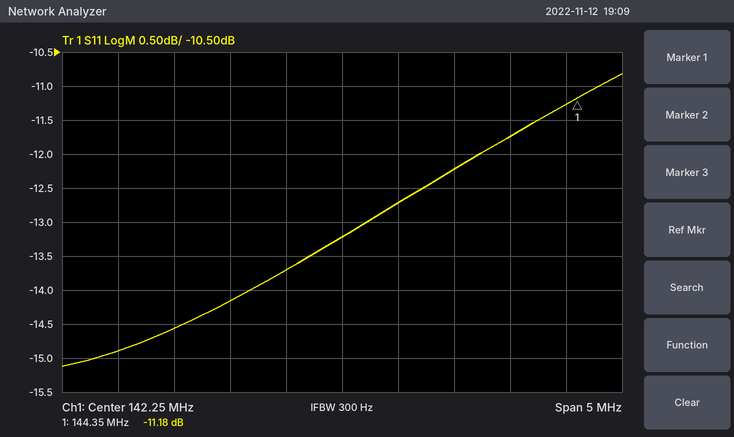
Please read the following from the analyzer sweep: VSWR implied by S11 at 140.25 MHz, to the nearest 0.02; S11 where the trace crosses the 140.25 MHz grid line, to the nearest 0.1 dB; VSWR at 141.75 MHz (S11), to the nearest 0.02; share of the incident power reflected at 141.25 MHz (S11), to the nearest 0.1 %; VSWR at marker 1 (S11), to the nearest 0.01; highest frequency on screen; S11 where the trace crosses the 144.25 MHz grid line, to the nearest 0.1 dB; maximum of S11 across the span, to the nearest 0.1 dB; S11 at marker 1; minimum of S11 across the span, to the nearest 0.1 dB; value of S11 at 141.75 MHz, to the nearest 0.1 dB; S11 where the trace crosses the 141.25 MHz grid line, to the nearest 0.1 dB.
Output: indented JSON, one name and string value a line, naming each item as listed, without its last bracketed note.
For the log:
{
  "VSWR implied by S11 at 140.25 MHz, to the nearest 0.02": "1.44",
  "S11 where the trace crosses the 140.25 MHz grid line, to the nearest 0.1 dB": "-14.9 dB",
  "VSWR at 141.75 MHz (S11), to the nearest 0.02": "1.52",
  "share of the incident power reflected at 141.25 MHz (S11), to the nearest 0.1 %": "3.8 %",
  "VSWR at marker 1 (S11), to the nearest 0.01": "1.76",
  "highest frequency on screen": "144.75 MHz",
  "S11 where the trace crosses the 144.25 MHz grid line, to the nearest 0.1 dB": "-11.3 dB",
  "maximum of S11 across the span, to the nearest 0.1 dB": "-10.8 dB",
  "S11 at marker 1": "-11.18 dB",
  "minimum of S11 across the span, to the nearest 0.1 dB": "-15.1 dB",
  "value of S11 at 141.75 MHz, to the nearest 0.1 dB": "-13.7 dB",
  "S11 where the trace crosses the 141.25 MHz grid line, to the nearest 0.1 dB": "-14.2 dB"
}
